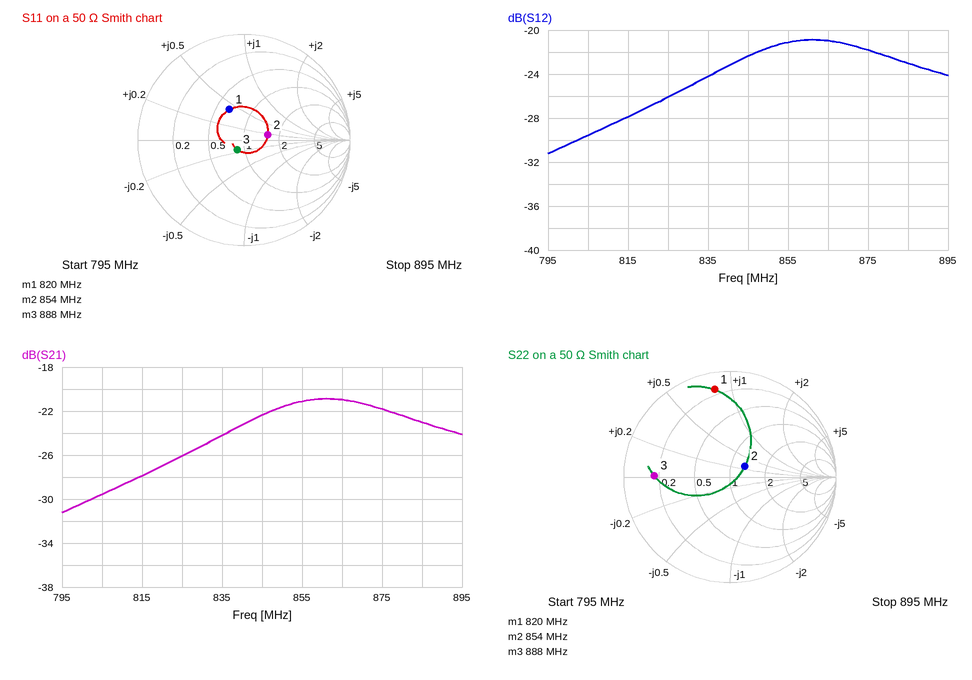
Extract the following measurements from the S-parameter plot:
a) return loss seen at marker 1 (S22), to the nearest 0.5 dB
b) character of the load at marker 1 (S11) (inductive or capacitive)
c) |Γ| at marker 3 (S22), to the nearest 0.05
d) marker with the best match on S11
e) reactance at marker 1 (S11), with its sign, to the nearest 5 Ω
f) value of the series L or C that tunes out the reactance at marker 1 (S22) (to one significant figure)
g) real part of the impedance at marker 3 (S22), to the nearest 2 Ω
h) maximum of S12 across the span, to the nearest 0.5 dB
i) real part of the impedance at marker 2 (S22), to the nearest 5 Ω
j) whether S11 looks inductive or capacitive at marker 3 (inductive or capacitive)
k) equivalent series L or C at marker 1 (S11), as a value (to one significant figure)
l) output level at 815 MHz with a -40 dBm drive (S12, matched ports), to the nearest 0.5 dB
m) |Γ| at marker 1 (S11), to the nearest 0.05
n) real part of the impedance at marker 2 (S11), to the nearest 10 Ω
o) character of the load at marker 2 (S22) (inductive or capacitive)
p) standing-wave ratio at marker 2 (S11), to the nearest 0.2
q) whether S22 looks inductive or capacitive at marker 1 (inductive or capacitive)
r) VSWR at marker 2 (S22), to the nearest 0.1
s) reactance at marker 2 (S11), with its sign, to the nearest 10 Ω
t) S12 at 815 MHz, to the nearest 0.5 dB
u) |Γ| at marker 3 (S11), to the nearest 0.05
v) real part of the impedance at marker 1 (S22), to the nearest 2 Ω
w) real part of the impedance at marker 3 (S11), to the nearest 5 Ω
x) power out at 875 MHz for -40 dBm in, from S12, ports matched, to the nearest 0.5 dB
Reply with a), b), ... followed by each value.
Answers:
a) 1.5 dB
b) inductive
c) 0.70
d) marker 3
e) +20 Ω
f) 5 pF
g) 8 Ω
h) -21.0 dB
i) 65 Ω
j) capacitive
k) 4 nH
l) -68.0 dBm
m) 0.30
n) 80 Ω
o) inductive
p) 1.6
q) inductive
r) 1.4
s) +10 Ω
t) -28.0 dB
u) 0.10
v) 8 Ω
w) 45 Ω
x) -62.0 dBm
